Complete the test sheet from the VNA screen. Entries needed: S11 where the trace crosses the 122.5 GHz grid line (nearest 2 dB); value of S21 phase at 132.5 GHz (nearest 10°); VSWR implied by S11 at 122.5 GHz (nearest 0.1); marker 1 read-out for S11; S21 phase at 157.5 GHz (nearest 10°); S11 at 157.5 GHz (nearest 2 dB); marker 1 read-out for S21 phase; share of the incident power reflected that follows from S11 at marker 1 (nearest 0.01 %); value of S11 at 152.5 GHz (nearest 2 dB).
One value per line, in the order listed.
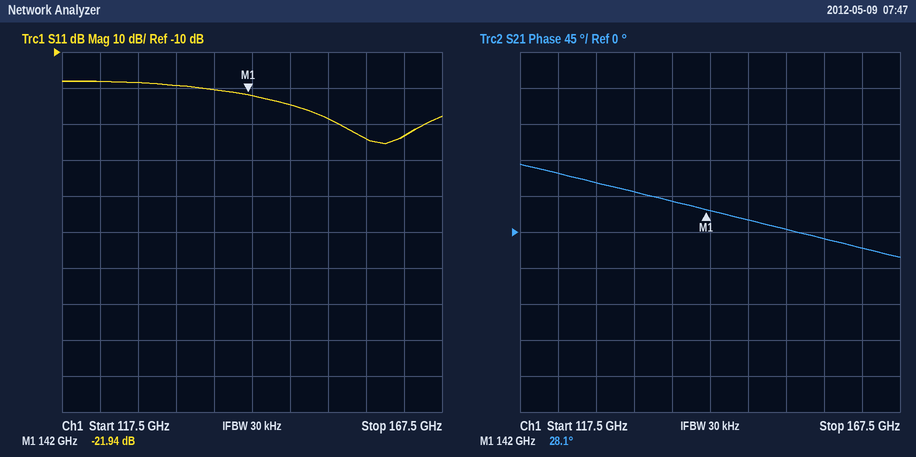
-18 dB
50°
1.3
-21.94 dB
-10°
-34 dB
28.1°
0.64 %
-28 dB
